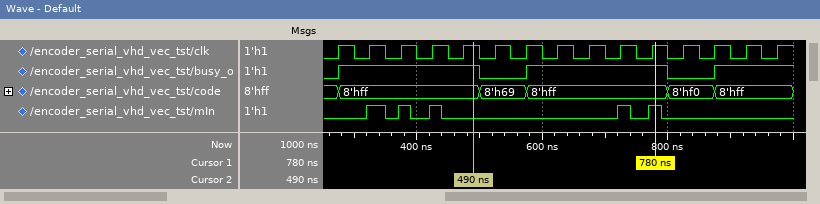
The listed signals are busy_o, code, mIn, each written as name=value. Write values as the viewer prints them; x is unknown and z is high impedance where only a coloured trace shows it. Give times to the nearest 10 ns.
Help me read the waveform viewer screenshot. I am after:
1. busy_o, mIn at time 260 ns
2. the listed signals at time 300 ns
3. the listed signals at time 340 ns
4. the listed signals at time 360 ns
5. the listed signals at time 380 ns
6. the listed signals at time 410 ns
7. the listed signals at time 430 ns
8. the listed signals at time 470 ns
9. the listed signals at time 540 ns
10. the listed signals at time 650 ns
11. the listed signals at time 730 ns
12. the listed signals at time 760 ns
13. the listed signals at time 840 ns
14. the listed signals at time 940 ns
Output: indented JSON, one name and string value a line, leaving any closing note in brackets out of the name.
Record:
{
  "busy_o, mIn at time 260 ns": "busy_o=0, mIn=0",
  "the listed signals at time 300 ns": "busy_o=1, code=8'hff, mIn=0",
  "the listed signals at time 340 ns": "busy_o=1, code=8'hff, mIn=1",
  "the listed signals at time 360 ns": "busy_o=1, code=8'hff, mIn=0",
  "the listed signals at time 380 ns": "busy_o=1, code=8'hff, mIn=1",
  "the listed signals at time 410 ns": "busy_o=1, code=8'hff, mIn=0",
  "the listed signals at time 430 ns": "busy_o=1, code=8'hff, mIn=1",
  "the listed signals at time 470 ns": "busy_o=1, code=8'hff, mIn=0",
  "the listed signals at time 540 ns": "busy_o=0, code=8'h69, mIn=0",
  "the listed signals at time 650 ns": "busy_o=1, code=8'hff, mIn=0",
  "the listed signals at time 730 ns": "busy_o=1, code=8'hff, mIn=1",
  "the listed signals at time 760 ns": "busy_o=1, code=8'hff, mIn=0",
  "the listed signals at time 840 ns": "busy_o=0, code=8'hf0, mIn=0",
  "the listed signals at time 940 ns": "busy_o=1, code=8'hff, mIn=0"
}
